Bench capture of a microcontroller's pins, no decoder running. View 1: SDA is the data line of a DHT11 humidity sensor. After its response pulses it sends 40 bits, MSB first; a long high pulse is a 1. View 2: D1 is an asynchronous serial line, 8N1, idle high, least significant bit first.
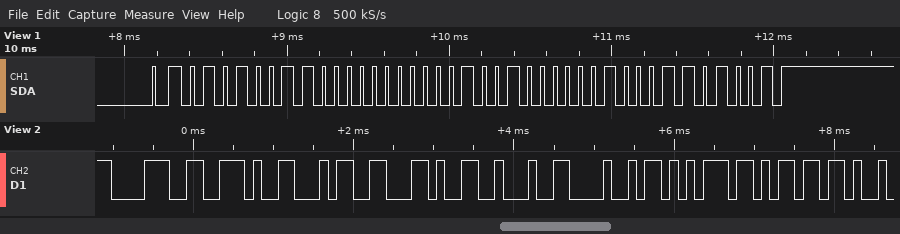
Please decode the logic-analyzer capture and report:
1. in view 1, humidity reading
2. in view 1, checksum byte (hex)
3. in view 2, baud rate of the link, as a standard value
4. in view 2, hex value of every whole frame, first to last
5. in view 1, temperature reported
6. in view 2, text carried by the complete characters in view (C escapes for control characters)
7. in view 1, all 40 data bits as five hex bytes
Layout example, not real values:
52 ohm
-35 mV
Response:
83 %
0x69
9600 baud
38 2E 34 2C 22 48 75 6D
18.4 °C
"8.4,\"Hum"
53 00 12 04 69
